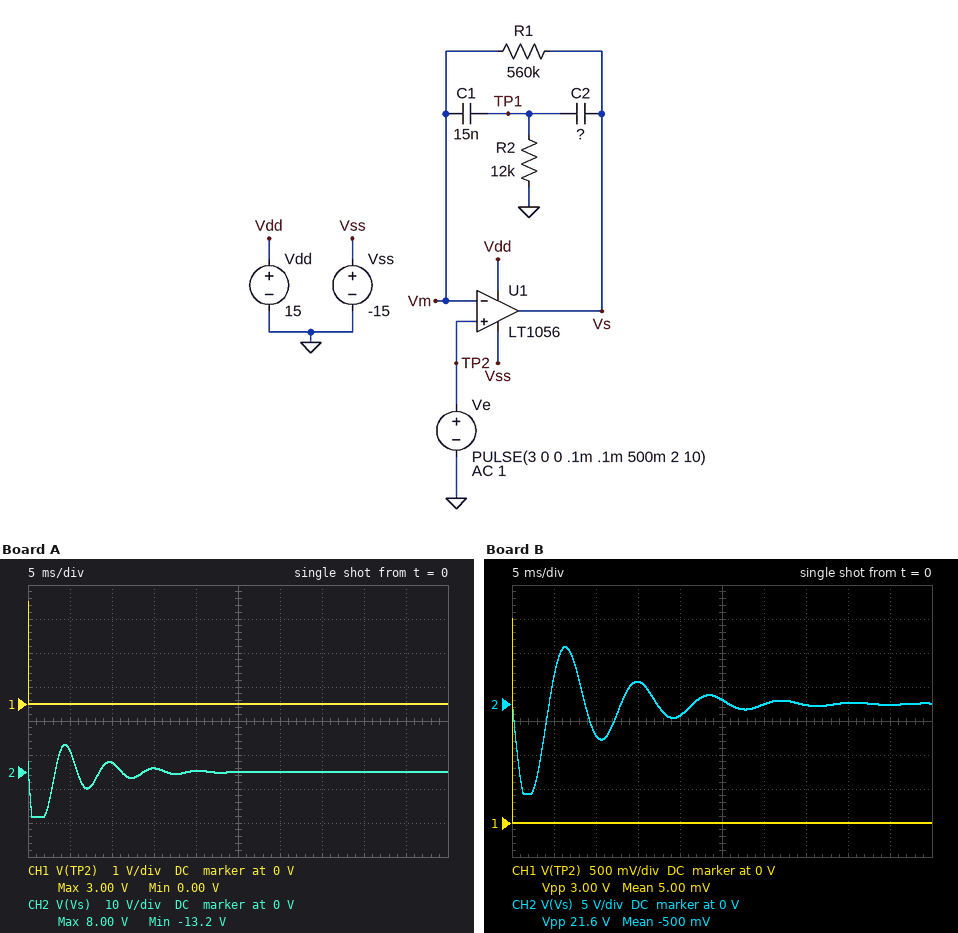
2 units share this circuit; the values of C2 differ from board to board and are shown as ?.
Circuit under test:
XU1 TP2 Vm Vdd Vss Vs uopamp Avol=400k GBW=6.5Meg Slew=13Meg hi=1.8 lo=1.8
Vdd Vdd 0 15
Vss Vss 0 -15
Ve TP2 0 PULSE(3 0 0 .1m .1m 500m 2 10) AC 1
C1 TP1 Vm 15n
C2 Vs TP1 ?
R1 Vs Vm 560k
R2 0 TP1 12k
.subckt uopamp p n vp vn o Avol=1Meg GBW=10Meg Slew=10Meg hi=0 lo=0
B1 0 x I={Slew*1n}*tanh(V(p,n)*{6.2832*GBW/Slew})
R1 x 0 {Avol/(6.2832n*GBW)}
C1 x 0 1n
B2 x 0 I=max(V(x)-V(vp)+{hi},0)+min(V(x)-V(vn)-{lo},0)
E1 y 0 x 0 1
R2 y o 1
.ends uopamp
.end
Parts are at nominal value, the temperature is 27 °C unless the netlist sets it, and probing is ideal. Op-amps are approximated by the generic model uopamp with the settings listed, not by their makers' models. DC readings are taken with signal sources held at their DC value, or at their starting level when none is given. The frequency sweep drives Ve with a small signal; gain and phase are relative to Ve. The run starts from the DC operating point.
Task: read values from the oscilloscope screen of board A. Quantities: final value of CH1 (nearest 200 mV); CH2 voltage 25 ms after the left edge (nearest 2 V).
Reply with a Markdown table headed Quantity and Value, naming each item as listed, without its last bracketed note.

| Quantity | Value |
|---|---|
| final value of CH1 | 0 V |
| CH2 voltage 25 ms after the left edge | 0 V |
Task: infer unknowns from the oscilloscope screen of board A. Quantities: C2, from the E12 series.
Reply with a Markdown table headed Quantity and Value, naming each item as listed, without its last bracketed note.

| Quantity | Value |
|---|---|
| C2, from the E12 series | 6.8 nF |
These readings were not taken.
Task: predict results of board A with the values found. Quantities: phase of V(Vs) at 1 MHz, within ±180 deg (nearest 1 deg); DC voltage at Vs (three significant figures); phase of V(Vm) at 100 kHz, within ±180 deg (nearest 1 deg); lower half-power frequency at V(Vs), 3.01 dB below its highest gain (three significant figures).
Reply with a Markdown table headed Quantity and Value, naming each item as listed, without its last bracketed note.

| Quantity | Value |
|---|---|
| phase of V(Vs) at 1 MHz, within ±180 deg | -9 deg |
| DC voltage at Vs | 3.00 V |
| phase of V(Vm) at 100 kHz, within ±180 deg | -1 deg |
| lower half-power frequency at V(Vs), 3.01 dB below its highest gain | 164 Hz |
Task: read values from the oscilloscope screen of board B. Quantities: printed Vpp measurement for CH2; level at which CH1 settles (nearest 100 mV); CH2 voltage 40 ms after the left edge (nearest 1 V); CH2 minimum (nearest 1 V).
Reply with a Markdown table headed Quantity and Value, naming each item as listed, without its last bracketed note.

| Quantity | Value |
|---|---|
| printed Vpp measurement for CH2 | 21.6 V |
| level at which CH1 settles | 0 V |
| CH2 voltage 40 ms after the left edge | 0 V |
| CH2 minimum | -13 V |
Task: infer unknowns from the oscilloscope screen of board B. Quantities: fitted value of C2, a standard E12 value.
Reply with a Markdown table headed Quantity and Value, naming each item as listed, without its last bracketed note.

| Quantity | Value |
|---|---|
| fitted value of C2, a standard E12 value | 18 nF |
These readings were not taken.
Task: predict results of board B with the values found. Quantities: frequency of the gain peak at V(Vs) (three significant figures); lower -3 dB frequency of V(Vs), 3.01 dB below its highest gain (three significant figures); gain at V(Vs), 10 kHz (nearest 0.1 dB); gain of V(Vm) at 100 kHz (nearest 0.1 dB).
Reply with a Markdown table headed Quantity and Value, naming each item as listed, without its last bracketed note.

| Quantity | Value |
|---|---|
| frequency of the gain peak at V(Vs) | 118 Hz |
| lower -3 dB frequency of V(Vs), 3.01 dB below its highest gain | 102 Hz |
| gain at V(Vs), 10 kHz | 0 dB |
| gain of V(Vm) at 100 kHz | 0 dB |
